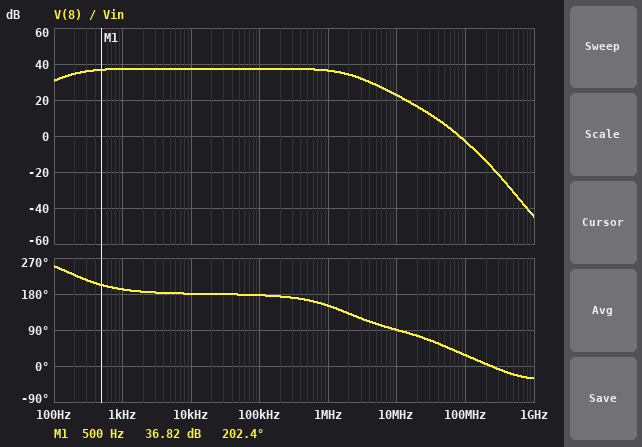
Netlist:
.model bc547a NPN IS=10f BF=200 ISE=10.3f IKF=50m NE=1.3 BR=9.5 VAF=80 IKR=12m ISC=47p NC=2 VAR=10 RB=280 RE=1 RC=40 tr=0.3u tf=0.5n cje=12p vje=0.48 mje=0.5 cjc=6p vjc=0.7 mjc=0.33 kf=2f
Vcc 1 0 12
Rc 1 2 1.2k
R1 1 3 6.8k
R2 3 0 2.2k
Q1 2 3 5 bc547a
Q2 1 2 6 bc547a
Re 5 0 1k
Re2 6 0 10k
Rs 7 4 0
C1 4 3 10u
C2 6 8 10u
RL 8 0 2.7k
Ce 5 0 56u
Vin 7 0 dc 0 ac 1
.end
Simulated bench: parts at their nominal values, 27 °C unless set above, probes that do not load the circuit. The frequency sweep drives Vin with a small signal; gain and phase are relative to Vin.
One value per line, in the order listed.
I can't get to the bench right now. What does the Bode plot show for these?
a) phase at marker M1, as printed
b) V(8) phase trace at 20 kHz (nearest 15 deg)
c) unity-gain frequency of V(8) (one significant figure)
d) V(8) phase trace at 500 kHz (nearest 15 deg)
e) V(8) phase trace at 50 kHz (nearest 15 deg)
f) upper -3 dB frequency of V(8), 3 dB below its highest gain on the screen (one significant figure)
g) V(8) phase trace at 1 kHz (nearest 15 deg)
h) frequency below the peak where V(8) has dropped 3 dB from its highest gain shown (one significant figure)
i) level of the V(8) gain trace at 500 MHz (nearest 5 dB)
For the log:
202.4 deg
180 deg
80 MHz
165 deg
180 deg
2 MHz
195 deg
200 Hz
-30 dB
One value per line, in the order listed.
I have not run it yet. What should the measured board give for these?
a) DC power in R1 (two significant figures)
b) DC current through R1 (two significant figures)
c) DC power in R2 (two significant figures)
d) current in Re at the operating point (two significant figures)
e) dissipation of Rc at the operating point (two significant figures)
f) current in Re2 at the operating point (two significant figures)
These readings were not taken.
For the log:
12 mW
1.3 mA
3.8 mW
2.2 mA
5.9 mW
870 µA
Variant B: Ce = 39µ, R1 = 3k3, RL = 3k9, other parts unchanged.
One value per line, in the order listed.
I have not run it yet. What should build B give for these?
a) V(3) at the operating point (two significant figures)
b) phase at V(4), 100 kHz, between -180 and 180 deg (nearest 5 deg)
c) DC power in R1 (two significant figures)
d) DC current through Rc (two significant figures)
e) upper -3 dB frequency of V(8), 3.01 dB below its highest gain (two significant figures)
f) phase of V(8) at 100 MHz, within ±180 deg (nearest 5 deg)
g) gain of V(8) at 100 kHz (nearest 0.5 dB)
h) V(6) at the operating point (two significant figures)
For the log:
4.8 V
0 deg
16 mW
4.0 mA
1.1 MHz
35 deg
40.5 dB
6.5 V
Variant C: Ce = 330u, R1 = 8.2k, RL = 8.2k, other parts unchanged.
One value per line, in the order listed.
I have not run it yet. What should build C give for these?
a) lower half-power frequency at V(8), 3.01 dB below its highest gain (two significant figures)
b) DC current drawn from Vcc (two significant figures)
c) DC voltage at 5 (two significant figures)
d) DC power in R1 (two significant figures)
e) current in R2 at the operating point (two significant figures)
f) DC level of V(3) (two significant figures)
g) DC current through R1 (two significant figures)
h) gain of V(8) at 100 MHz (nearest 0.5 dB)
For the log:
37 Hz
3.9 mA
1.8 V
11 mW
1.1 mA
2.5 V
1.2 mA
-3.0 dB
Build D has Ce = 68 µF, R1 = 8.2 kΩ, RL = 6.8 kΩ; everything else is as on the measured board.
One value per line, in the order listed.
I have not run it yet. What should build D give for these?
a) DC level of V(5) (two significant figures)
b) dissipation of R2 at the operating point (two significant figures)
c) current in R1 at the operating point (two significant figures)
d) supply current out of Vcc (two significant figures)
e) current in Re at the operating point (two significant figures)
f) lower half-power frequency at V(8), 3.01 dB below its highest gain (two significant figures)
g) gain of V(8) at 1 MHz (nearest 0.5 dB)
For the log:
1.8 V
2.9 mW
1.2 mA
3.9 mA
1.8 mA
140 Hz
35.5 dB
